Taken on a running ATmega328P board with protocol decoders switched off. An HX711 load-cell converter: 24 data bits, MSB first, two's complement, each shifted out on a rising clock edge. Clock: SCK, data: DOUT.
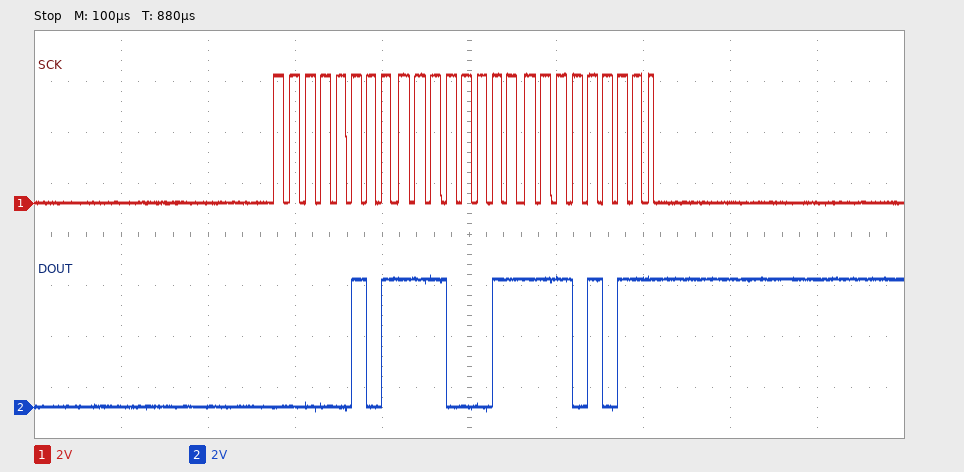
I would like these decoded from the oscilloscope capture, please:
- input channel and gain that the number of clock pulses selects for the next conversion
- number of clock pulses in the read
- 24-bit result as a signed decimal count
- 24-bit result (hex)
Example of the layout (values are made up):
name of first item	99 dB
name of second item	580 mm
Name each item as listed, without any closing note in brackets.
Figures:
input channel and gain that the number of clock pulses selects for the next conversion	channel A, gain 128
number of clock pulses in the read	25
24-bit result as a signed decimal count	386027
24-bit result	0x05E3EB
